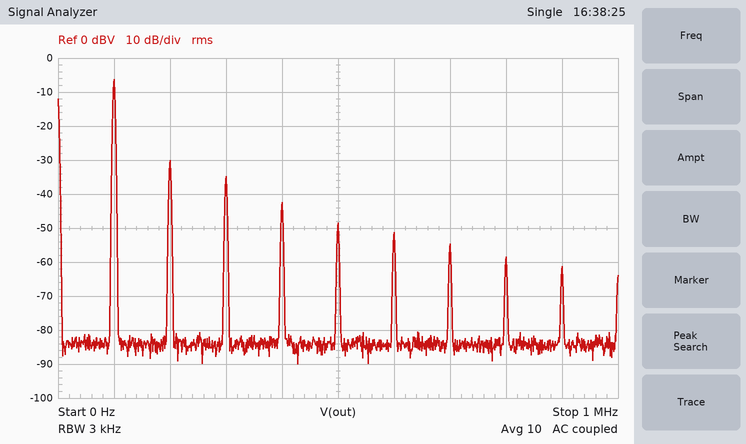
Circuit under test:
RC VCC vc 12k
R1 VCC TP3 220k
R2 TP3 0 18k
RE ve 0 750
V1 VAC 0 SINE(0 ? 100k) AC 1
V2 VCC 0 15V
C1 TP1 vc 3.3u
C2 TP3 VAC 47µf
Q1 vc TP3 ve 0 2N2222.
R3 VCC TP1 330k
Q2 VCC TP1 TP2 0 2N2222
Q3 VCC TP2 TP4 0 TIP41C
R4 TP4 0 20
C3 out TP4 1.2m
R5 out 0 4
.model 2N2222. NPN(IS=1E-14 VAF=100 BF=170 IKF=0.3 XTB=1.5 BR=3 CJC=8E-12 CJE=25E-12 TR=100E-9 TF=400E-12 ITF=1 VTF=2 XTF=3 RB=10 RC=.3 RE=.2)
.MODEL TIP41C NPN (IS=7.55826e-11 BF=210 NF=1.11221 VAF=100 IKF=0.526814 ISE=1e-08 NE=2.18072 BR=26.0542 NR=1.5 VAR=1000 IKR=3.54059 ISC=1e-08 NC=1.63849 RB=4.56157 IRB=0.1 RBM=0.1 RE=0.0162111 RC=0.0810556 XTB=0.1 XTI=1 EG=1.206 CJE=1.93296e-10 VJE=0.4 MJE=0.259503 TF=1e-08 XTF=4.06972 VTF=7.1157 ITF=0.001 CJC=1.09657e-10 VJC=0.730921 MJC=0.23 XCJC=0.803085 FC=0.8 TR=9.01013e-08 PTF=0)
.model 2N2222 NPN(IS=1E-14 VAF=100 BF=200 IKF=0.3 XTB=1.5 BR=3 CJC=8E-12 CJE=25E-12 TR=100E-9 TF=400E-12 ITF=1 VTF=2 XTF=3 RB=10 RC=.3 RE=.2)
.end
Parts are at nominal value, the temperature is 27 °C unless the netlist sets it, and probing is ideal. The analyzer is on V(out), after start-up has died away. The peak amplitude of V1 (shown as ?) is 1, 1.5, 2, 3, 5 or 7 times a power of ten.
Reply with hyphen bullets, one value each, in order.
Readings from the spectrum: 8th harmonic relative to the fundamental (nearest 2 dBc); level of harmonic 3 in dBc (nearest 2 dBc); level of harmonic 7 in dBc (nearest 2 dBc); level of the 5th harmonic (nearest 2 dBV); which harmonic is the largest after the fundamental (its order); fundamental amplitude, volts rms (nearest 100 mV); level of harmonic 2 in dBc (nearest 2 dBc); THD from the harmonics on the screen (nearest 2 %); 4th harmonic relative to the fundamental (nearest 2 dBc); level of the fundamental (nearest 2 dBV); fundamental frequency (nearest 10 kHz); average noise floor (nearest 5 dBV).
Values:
- -52 dBc
- -28 dBc
- -48 dBc
- -48 dBV
- 2
- 500 mV
- -24 dBc
- 8 %
- -36 dBc
- -6 dBV
- 100 kHz
- -85 dBV
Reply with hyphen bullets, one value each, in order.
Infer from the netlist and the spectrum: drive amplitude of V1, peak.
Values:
- 70 mV
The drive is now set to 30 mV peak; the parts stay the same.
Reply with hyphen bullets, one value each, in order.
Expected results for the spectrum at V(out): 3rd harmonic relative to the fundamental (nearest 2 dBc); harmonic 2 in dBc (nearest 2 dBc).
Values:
- -56 dBc
- -40 dBc
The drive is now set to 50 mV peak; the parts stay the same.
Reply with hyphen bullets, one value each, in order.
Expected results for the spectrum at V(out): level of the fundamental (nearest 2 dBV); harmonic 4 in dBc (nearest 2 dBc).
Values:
- -8 dBV
- -48 dBc
